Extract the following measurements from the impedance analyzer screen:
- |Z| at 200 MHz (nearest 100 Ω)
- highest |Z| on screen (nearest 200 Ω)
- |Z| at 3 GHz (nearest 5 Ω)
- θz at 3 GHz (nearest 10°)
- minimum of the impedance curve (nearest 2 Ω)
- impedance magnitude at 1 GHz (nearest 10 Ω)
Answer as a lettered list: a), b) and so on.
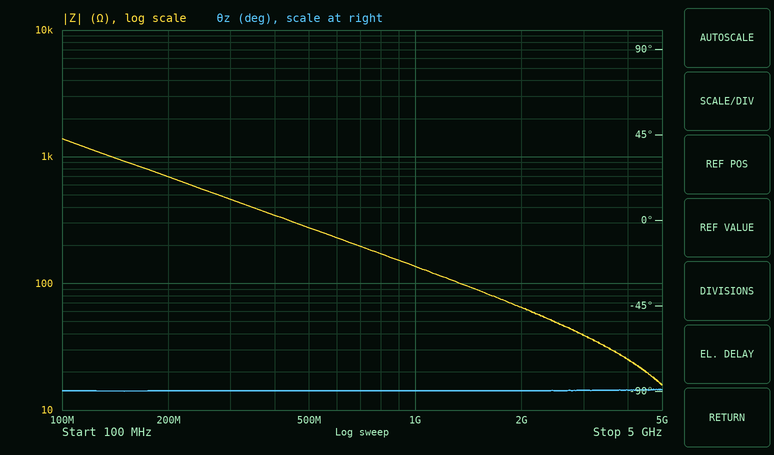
a) 700 Ω
b) 1.4 kΩ
c) 40 Ω
d) -90°
e) 16 Ω
f) 140 Ω
